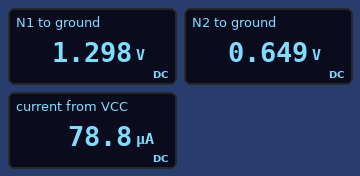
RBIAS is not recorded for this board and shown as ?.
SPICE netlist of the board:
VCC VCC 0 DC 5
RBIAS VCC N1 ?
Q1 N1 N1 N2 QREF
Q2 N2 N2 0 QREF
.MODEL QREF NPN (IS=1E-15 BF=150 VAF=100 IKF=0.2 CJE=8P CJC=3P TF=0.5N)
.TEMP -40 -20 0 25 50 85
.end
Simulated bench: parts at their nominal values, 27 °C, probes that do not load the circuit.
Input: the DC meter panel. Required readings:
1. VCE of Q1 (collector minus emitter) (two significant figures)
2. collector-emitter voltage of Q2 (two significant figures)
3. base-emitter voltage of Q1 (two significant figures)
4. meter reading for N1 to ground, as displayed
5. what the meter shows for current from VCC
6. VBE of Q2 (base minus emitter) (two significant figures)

650 mV
650 mV
650 mV
1.298 V
78.8 µA
650 mV
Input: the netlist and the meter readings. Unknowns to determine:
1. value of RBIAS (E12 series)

47 kΩ
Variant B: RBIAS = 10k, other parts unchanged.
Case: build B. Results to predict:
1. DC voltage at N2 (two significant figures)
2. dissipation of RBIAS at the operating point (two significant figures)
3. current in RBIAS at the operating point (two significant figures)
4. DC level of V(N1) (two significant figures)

690 mV
1.3 mW
360 µA
1.4 V
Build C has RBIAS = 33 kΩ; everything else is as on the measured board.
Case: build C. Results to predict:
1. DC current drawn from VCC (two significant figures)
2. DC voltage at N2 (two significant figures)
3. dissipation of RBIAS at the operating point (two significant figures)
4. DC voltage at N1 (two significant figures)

110 µA
660 mV
410 µW
1.3 V
